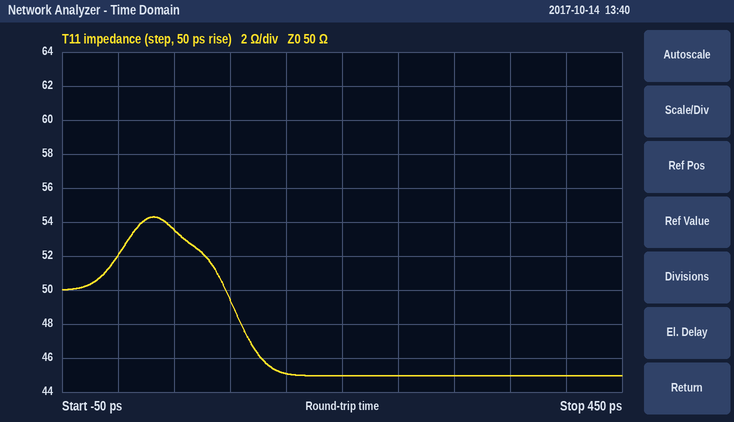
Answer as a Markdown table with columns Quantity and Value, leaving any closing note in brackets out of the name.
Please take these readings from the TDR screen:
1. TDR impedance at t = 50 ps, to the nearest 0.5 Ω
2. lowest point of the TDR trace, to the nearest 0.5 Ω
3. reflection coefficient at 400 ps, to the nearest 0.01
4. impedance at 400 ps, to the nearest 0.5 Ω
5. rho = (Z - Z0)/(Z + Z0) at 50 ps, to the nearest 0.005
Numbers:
| Quantity | Value |
|---|---|
| TDR impedance at t = 50 ps, to the nearest 0.5 Ω | 53.5 Ω |
| lowest point of the TDR trace, to the nearest 0.5 Ω | 45.0 Ω |
| reflection coefficient at 400 ps, to the nearest 0.01 | -0.05 |
| impedance at 400 ps, to the nearest 0.5 Ω | 45.0 Ω |
| rho = (Z - Z0)/(Z + Z0) at 50 ps, to the nearest 0.005 | +0.035 |
